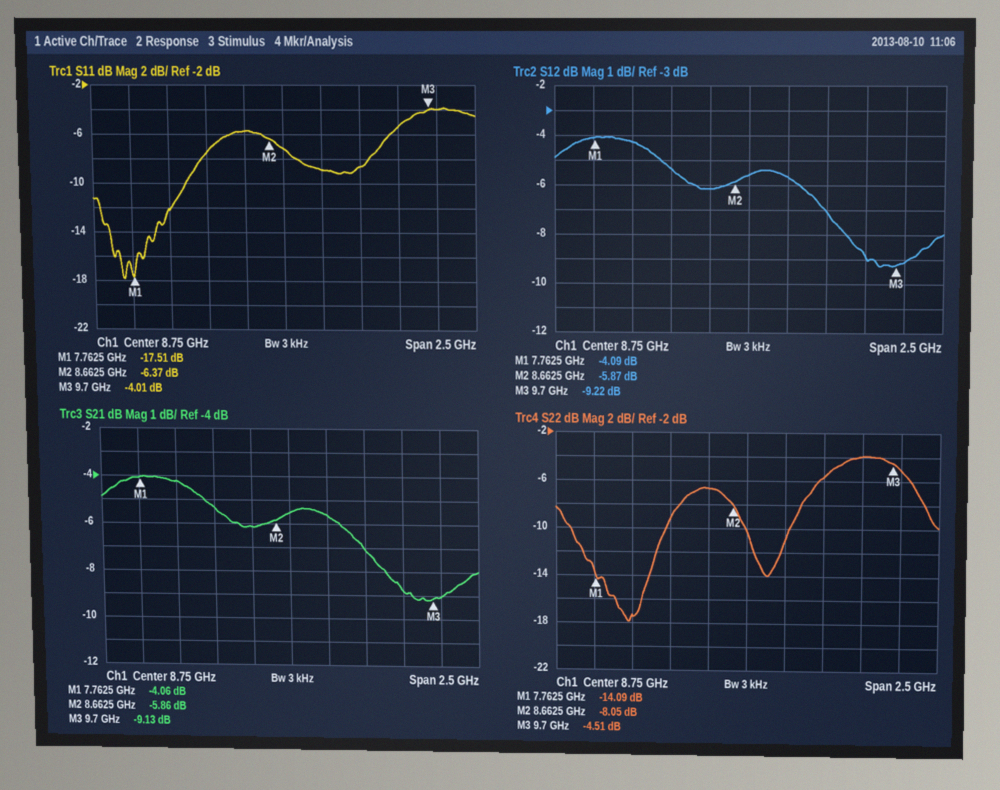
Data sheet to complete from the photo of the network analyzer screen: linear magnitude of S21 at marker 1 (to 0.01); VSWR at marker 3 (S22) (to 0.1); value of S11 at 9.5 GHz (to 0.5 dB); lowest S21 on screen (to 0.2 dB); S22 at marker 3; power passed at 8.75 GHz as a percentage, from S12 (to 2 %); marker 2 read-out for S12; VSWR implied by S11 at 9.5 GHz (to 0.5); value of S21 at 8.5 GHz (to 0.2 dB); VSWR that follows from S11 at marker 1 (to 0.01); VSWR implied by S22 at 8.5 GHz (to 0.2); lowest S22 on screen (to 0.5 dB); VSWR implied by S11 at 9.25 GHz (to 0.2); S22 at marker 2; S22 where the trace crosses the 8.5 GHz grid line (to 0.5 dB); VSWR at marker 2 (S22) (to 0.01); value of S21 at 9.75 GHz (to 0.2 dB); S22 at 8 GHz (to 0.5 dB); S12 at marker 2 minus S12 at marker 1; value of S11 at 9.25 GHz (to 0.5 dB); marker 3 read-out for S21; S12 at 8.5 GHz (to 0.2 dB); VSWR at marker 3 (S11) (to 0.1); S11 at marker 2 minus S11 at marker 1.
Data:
0.63
3.9
-5.5 dB
-9.2 dB
-4.51 dB
28 %
-5.87 dB
3.5
-6.2 dB
1.31
2.8
-18.0 dB
2.2
-8.05 dB
-6.5 dB
2.31
-9.0 dB
-17.5 dB
-1.78 dB
-8.5 dB
-9.13 dB
-6.2 dB
4.4
11.14 dB
